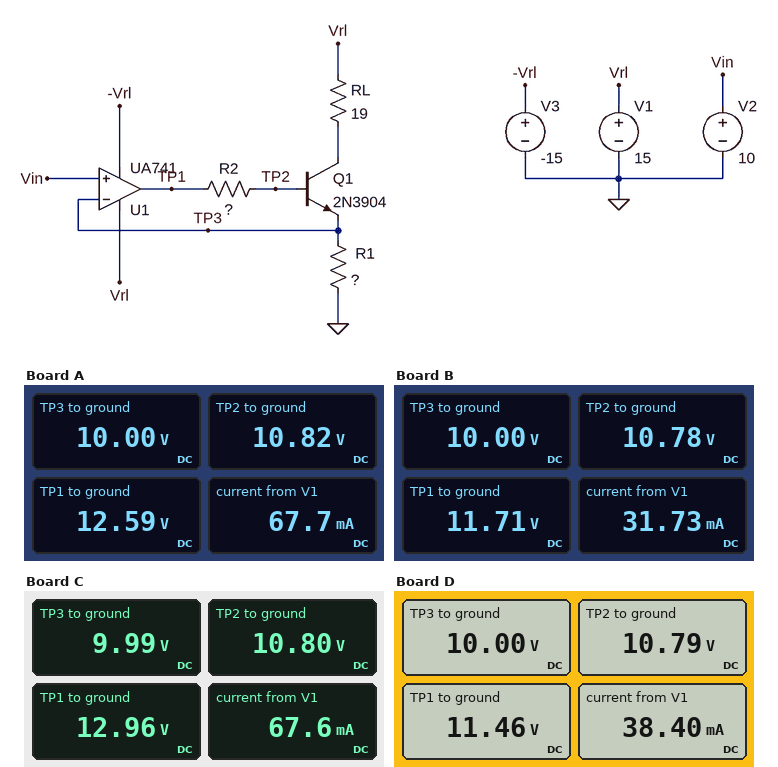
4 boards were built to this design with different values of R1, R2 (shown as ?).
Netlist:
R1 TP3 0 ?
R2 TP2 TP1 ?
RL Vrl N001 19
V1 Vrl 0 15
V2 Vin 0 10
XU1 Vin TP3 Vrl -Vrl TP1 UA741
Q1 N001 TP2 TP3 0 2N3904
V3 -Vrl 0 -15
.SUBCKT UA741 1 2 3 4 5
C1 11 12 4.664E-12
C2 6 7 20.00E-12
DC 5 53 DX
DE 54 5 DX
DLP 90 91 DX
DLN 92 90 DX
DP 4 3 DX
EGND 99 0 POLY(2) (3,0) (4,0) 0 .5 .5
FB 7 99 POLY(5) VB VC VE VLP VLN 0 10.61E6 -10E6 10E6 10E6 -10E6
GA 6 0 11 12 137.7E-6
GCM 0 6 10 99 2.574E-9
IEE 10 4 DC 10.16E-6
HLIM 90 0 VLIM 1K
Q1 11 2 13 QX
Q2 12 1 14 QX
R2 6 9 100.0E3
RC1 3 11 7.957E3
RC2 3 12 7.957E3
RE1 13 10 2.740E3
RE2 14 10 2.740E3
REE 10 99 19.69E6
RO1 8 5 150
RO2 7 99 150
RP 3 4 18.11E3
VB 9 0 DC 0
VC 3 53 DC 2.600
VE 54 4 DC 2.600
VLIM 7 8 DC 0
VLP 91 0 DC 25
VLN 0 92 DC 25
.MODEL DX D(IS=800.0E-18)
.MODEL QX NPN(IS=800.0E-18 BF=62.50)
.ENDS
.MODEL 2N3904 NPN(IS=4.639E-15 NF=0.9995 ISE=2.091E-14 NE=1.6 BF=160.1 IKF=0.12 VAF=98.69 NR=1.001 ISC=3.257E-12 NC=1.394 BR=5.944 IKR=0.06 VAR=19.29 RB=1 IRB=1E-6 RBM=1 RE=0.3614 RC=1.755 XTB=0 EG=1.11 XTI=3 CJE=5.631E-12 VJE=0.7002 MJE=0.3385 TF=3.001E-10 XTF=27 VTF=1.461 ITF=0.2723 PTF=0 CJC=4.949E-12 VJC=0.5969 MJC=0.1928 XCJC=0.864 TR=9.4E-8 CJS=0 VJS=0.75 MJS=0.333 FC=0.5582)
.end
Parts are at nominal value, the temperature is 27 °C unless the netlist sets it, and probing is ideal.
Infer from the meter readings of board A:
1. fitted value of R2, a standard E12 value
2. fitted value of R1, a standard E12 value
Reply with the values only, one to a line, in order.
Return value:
2.7 kΩ
150 Ω
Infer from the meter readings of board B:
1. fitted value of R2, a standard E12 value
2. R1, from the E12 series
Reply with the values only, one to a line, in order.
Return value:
3.9 kΩ
330 Ω
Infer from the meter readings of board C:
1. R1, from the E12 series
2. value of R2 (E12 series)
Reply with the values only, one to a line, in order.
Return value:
150 Ω
3.3 kΩ
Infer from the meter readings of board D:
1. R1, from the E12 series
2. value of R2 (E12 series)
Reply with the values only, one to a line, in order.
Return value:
270 Ω
2.2 kΩ
